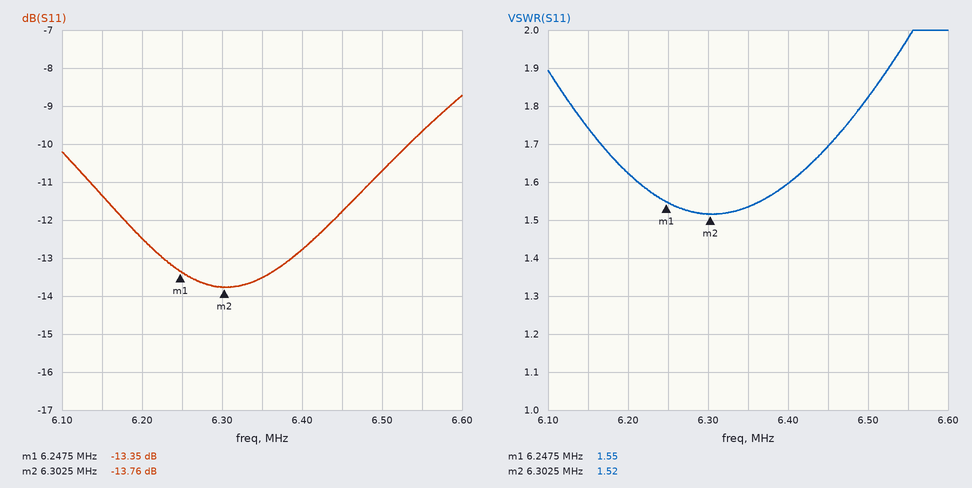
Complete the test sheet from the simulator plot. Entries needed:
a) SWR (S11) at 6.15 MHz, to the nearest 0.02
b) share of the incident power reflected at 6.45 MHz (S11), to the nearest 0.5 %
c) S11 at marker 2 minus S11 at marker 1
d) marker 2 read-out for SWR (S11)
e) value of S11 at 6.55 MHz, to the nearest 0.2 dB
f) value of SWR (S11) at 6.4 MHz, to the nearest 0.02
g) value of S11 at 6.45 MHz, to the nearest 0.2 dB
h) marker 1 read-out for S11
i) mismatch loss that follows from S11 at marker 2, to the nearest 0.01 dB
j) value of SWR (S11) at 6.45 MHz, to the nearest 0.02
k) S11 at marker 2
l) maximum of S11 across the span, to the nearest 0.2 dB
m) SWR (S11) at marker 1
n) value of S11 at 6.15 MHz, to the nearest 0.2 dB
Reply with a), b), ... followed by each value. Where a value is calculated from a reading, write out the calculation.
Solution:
a) 1.74
b) 10^(-11.8/10) ≈ 6.61 %, so 6.5 % to the nearest 0.5 %
c) -13.76 − (-13.35) = -0.41 dB
d) 1.52
e) -9.6 dB
f) 1.60
g) -11.8 dB
h) -13.35 dB
i) −10 log10(1 − 10^(-13.76/10)) ≈ 0.19 dB
j) 1.70
k) -13.76 dB
l) -8.8 dB
m) 1.55
n) -11.4 dB
